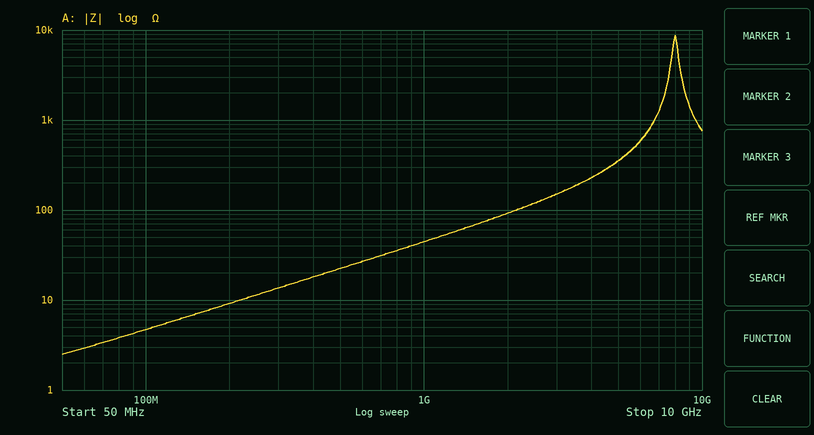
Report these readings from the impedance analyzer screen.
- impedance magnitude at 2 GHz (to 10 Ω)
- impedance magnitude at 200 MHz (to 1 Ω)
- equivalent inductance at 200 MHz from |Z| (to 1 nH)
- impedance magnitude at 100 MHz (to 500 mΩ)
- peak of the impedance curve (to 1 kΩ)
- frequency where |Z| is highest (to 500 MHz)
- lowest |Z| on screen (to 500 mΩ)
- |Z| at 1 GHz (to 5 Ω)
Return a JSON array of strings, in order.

["90 Ω", "9 Ω", "7 nH", "4.5 Ω", "9 kΩ", "8.0 GHz", "2.5 Ω", "45 Ω"]
